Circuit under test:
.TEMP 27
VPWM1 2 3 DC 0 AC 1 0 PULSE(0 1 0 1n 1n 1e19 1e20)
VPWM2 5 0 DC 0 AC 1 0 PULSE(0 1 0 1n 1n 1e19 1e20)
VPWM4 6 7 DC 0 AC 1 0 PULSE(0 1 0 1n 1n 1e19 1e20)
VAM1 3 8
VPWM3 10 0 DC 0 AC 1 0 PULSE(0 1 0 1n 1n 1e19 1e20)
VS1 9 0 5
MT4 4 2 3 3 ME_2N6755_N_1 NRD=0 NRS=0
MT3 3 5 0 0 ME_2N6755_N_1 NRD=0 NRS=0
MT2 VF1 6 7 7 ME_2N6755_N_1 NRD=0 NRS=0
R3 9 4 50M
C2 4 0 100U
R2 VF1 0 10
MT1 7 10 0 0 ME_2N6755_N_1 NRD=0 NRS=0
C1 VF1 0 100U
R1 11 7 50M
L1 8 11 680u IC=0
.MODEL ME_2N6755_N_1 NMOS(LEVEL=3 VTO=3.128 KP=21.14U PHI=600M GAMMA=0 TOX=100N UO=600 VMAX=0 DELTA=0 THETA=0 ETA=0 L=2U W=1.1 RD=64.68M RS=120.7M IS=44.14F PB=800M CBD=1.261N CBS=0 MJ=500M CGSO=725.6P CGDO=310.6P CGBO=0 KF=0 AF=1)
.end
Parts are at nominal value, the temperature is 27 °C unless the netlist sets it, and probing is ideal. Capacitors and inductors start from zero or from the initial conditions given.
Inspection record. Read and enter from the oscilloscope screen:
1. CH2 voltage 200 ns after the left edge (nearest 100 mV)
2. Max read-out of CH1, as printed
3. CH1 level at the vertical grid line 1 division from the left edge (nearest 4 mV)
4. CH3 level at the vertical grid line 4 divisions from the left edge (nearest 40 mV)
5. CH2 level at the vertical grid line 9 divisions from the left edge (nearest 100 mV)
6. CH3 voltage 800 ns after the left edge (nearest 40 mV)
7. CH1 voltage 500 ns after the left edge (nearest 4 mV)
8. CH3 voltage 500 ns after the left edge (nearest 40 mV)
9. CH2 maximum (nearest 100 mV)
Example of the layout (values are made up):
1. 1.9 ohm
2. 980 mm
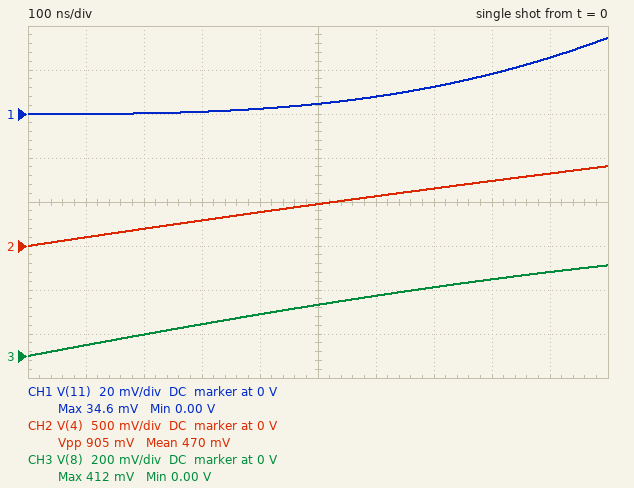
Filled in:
1. 200 mV
2. 34.6 mV
3. 0 V
4. 200 mV
5. 800 mV
6. 360 mV
7. 4 mV
8. 240 mV
9. 900 mV
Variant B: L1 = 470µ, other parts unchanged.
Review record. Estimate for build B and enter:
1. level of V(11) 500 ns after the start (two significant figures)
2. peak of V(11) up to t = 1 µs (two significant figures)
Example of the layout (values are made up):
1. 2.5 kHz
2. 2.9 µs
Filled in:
1. 6.6 mV
2. 49 mV
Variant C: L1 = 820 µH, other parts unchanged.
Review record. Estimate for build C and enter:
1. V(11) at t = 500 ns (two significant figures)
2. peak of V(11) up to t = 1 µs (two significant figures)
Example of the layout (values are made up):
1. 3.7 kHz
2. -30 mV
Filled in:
1. 3.8 mV
2. 29 mV
